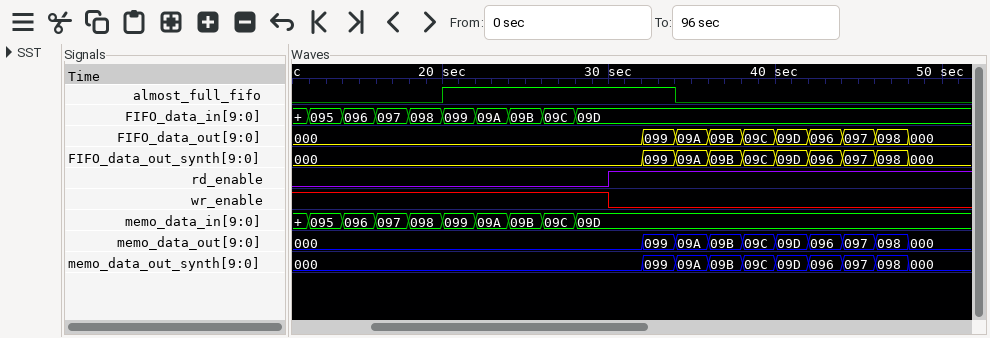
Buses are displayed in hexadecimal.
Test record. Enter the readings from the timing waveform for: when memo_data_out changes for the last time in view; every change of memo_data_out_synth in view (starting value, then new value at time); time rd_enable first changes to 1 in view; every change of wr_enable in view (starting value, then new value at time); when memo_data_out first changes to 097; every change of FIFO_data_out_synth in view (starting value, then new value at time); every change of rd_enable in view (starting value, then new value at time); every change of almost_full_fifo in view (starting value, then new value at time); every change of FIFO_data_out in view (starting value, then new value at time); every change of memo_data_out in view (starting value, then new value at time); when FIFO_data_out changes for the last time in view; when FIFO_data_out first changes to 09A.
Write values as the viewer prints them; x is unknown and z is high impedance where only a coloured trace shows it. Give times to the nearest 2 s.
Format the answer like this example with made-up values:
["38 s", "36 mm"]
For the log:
["48 s", "000, 099 at 32 s, 09A at 34 s, 09B at 36 s, 09C at 38 s, 09D at 40 s, 096 at 42 s, 097 at 44 s, 098 at 46 s, 000 at 48 s", "30 s", "1, 0 at 30 s", "44 s", "000, 099 at 32 s, 09A at 34 s, 09B at 36 s, 09C at 38 s, 09D at 40 s, 096 at 42 s, 097 at 44 s, 098 at 46 s, 000 at 48 s", "0, 1 at 30 s", "0, 1 at 20 s, 0 at 34 s", "000, 099 at 32 s, 09A at 34 s, 09B at 36 s, 09C at 38 s, 09D at 40 s, 096 at 42 s, 097 at 44 s, 098 at 46 s, 000 at 48 s", "000, 099 at 32 s, 09A at 34 s, 09B at 36 s, 09C at 38 s, 09D at 40 s, 096 at 42 s, 097 at 44 s, 098 at 46 s, 000 at 48 s", "48 s", "34 s"]
